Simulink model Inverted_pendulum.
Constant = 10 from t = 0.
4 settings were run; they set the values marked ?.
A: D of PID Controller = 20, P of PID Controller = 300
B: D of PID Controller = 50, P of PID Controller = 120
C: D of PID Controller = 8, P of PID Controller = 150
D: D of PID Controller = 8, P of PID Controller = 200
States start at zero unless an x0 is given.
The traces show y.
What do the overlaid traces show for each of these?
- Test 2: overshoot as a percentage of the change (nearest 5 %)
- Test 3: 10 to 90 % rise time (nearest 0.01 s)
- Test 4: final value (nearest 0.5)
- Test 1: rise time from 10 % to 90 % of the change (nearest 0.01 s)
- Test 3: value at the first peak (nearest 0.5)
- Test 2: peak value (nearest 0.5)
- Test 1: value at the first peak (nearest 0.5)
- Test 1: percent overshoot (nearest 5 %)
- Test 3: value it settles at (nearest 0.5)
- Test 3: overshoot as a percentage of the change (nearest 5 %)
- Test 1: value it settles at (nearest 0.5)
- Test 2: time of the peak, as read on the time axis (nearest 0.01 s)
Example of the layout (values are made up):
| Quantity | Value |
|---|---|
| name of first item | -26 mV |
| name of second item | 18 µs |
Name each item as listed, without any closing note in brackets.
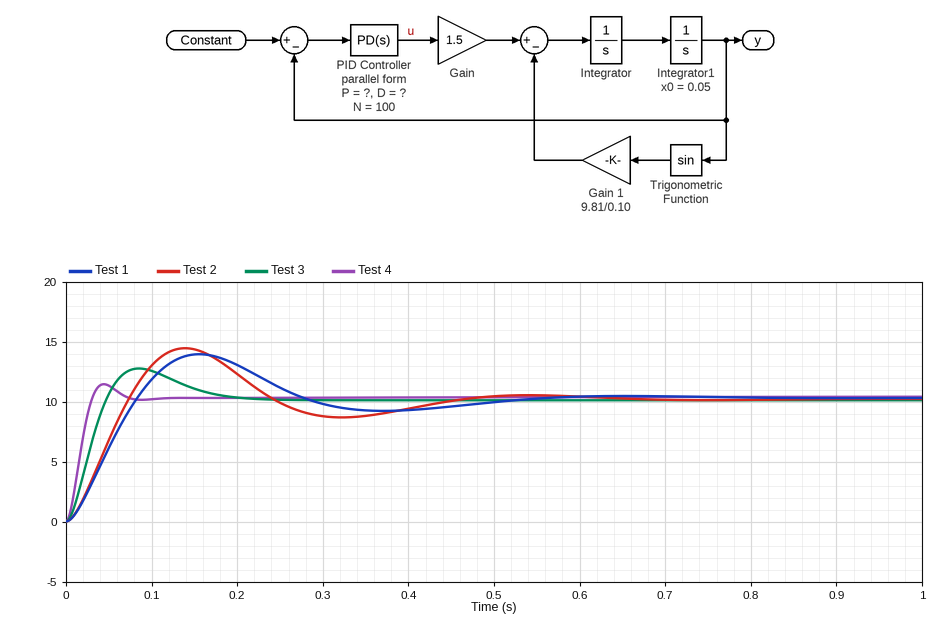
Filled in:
| Quantity | Value |
|---|---|
| Test 2: overshoot as a percentage of the change | 40 % |
| Test 3: 10 to 90 % rise time | 0.03 s |
| Test 4: final value | 10.5 |
| Test 1: rise time from 10 % to 90 % of the change | 0.06 s |
| Test 3: value at the first peak | 13.0 |
| Test 2: peak value | 14.5 |
| Test 1: value at the first peak | 14.0 |
| Test 1: percent overshoot | 35 % |
| Test 3: value it settles at | 10.0 |
| Test 3: overshoot as a percentage of the change | 25 % |
| Test 1: value it settles at | 10.5 |
| Test 2: time of the peak, as read on the time axis | 0.14 s |
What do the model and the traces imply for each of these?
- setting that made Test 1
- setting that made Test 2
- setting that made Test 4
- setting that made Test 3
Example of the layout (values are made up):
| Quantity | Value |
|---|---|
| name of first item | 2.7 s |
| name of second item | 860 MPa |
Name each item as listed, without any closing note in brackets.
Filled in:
| Quantity | Value |
|---|---|
| setting that made Test 1 | C |
| setting that made Test 2 | D |
| setting that made Test 4 | B |
| setting that made Test 3 | A |
